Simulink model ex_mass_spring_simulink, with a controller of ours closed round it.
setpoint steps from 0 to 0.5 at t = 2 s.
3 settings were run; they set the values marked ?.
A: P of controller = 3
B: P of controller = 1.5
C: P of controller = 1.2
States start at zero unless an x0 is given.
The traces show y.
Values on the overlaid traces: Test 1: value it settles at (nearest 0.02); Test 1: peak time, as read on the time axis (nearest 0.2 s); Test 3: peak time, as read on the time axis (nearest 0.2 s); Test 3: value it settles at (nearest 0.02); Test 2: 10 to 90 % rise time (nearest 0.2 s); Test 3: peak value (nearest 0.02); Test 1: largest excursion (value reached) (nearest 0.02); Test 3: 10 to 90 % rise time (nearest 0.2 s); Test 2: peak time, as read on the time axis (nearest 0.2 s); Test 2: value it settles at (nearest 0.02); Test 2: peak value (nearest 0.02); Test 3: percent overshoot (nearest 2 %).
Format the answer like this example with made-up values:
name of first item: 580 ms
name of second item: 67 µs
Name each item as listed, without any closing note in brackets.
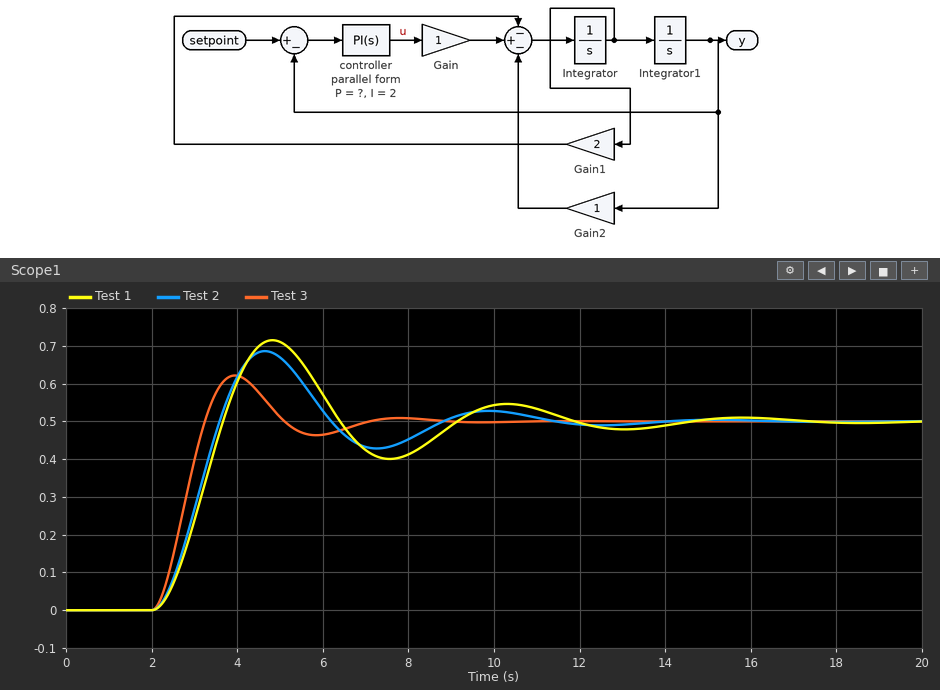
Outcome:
Test 1: value it settles at: 0.50
Test 1: peak time, as read on the time axis: 4.8 s
Test 3: peak time, as read on the time axis: 4.0 s
Test 3: value it settles at: 0.50
Test 2: 10 to 90 % rise time: 1.0 s
Test 3: peak value: 0.62
Test 1: largest excursion (value reached): 0.72
Test 3: 10 to 90 % rise time: 0.8 s
Test 2: peak time, as read on the time axis: 4.6 s
Test 2: value it settles at: 0.50
Test 2: peak value: 0.68
Test 3: percent overshoot: 24 %
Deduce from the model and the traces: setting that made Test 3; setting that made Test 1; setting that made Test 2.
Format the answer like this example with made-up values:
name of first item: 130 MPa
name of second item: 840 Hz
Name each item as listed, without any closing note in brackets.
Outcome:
setting that made Test 3: A
setting that made Test 1: C
setting that made Test 2: B
